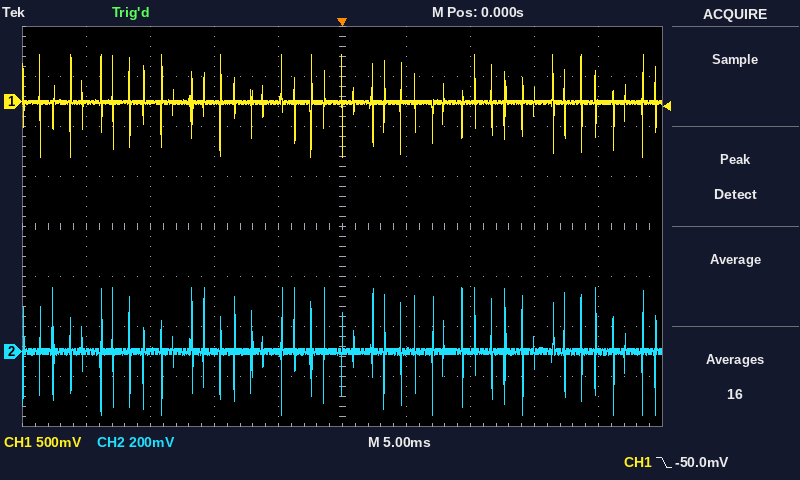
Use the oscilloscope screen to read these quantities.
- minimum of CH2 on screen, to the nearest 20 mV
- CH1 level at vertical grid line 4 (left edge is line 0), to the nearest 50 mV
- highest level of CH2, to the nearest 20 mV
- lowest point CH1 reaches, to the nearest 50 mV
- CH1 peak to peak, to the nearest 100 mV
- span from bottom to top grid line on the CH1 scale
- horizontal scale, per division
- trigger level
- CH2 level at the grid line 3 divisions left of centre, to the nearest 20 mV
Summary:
-260 mV
50 mV
260 mV
-550 mV
1.00 V
4 V
5 ms
-50.0 mV
0 mV
